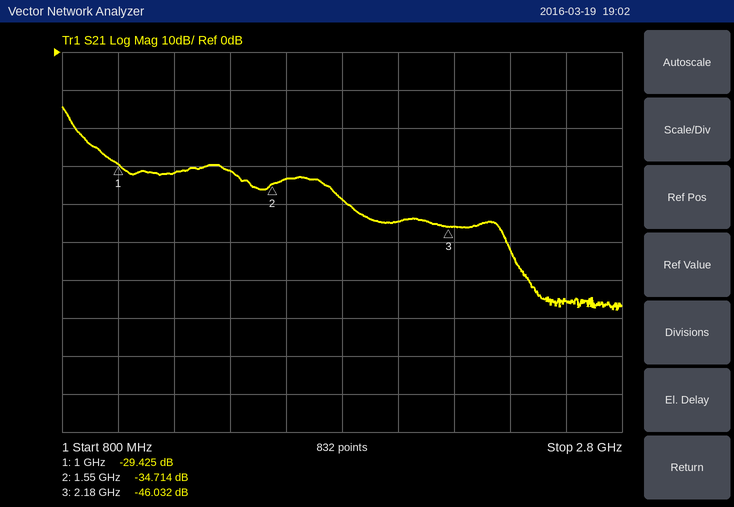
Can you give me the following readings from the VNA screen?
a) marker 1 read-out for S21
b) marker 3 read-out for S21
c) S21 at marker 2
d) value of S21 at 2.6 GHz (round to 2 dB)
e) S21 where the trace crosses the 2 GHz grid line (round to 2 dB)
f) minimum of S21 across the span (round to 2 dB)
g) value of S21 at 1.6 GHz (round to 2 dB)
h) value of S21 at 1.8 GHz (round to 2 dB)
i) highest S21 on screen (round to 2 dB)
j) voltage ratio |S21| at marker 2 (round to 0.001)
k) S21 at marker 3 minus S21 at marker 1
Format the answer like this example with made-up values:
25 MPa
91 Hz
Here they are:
-29.425 dB
-46.032 dB
-34.714 dB
-66 dB
-44 dB
-68 dB
-34 dB
-38 dB
-14 dB
0.018
-16.607 dB
